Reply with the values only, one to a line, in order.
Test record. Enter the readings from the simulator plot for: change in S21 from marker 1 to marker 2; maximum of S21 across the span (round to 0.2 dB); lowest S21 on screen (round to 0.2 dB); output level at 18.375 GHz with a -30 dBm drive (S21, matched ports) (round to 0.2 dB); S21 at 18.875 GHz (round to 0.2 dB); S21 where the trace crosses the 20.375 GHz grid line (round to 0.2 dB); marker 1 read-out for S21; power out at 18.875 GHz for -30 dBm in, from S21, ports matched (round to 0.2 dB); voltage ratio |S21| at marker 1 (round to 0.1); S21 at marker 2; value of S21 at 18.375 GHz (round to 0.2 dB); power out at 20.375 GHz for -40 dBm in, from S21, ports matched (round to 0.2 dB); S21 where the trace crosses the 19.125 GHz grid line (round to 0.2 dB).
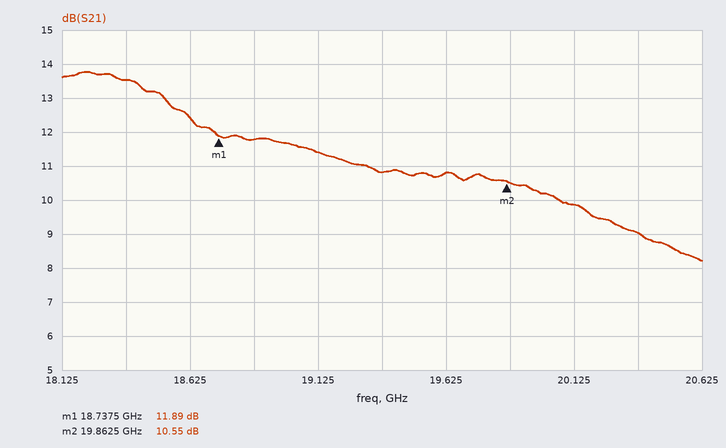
-1.34 dB
13.8 dB
8.2 dB
-16.4 dBm
11.8 dB
9.0 dB
11.89 dB
-18.2 dBm
3.9
10.55 dB
13.6 dB
-31.0 dBm
11.4 dB
